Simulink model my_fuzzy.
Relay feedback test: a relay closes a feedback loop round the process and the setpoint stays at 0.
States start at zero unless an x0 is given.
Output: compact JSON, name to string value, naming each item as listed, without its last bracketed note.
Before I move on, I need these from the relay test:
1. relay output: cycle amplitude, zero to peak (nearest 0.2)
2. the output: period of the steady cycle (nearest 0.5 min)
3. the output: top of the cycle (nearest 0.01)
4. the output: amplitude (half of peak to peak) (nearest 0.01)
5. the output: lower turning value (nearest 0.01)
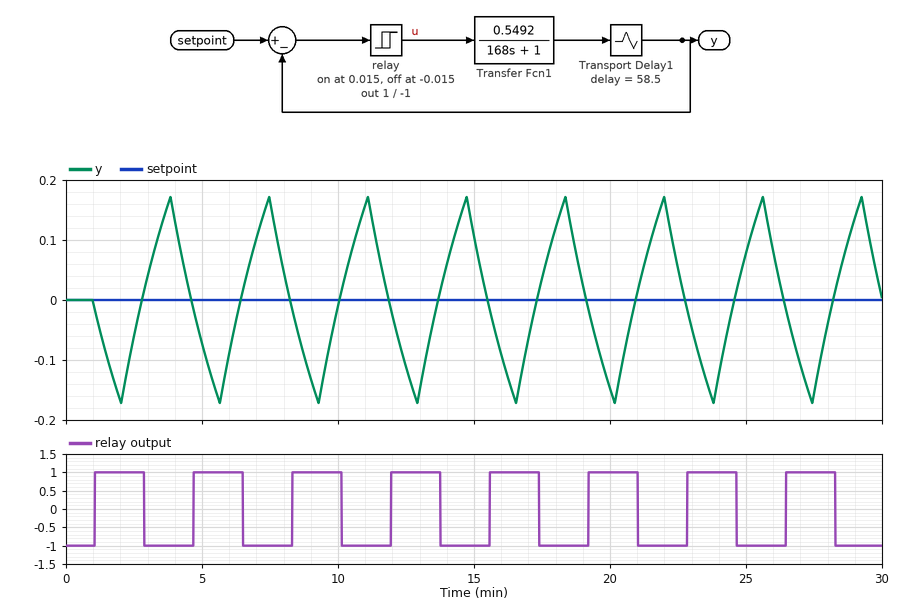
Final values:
{"relay output: cycle amplitude, zero to peak": "1.0", "the output: period of the steady cycle": "3.5 min", "the output: top of the cycle": "0.17", "the output: amplitude (half of peak to peak)": "0.17", "the output: lower turning value": "-0.17"}
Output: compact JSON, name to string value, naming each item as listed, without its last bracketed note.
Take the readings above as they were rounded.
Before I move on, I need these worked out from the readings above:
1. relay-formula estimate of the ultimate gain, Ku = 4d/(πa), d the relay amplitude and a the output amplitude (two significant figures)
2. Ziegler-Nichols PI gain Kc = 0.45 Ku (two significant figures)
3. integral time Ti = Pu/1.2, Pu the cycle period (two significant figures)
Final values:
{"relay-formula estimate of the ultimate gain, Ku = 4d/(πa), d the relay amplitude and a the output amplitude": "7.5", "Ziegler-Nichols PI gain Kc = 0.45 Ku": "3.4", "integral time Ti = Pu/1.2, Pu the cycle period": "2.9 min"}
